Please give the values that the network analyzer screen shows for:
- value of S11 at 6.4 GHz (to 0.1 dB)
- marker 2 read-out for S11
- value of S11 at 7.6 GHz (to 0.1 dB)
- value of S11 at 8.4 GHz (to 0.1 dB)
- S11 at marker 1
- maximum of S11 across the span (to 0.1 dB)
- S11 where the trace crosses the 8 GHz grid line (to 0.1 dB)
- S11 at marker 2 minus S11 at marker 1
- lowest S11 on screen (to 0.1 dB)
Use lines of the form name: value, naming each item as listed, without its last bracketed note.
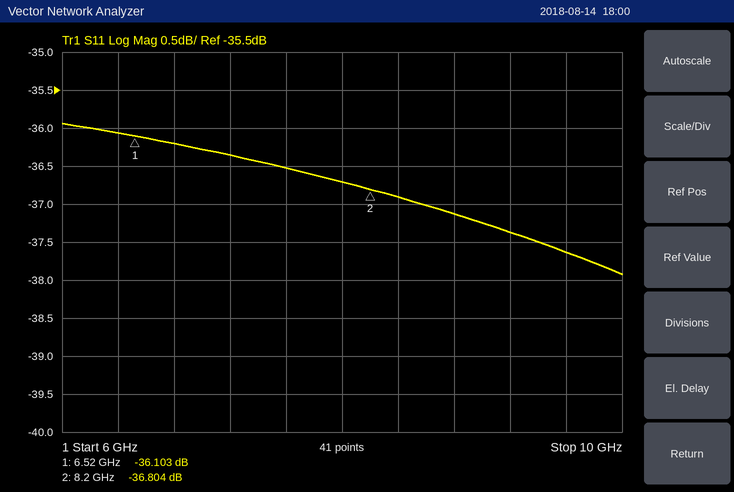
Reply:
value of S11 at 6.4 GHz: -36.1 dB
marker 2 read-out for S11: -36.804 dB
value of S11 at 7.6 GHz: -36.5 dB
value of S11 at 8.4 GHz: -36.9 dB
S11 at marker 1: -36.103 dB
maximum of S11 across the span: -35.9 dB
S11 where the trace crosses the 8 GHz grid line: -36.7 dB
S11 at marker 2 minus S11 at marker 1: -0.701 dB
lowest S11 on screen: -37.9 dB
